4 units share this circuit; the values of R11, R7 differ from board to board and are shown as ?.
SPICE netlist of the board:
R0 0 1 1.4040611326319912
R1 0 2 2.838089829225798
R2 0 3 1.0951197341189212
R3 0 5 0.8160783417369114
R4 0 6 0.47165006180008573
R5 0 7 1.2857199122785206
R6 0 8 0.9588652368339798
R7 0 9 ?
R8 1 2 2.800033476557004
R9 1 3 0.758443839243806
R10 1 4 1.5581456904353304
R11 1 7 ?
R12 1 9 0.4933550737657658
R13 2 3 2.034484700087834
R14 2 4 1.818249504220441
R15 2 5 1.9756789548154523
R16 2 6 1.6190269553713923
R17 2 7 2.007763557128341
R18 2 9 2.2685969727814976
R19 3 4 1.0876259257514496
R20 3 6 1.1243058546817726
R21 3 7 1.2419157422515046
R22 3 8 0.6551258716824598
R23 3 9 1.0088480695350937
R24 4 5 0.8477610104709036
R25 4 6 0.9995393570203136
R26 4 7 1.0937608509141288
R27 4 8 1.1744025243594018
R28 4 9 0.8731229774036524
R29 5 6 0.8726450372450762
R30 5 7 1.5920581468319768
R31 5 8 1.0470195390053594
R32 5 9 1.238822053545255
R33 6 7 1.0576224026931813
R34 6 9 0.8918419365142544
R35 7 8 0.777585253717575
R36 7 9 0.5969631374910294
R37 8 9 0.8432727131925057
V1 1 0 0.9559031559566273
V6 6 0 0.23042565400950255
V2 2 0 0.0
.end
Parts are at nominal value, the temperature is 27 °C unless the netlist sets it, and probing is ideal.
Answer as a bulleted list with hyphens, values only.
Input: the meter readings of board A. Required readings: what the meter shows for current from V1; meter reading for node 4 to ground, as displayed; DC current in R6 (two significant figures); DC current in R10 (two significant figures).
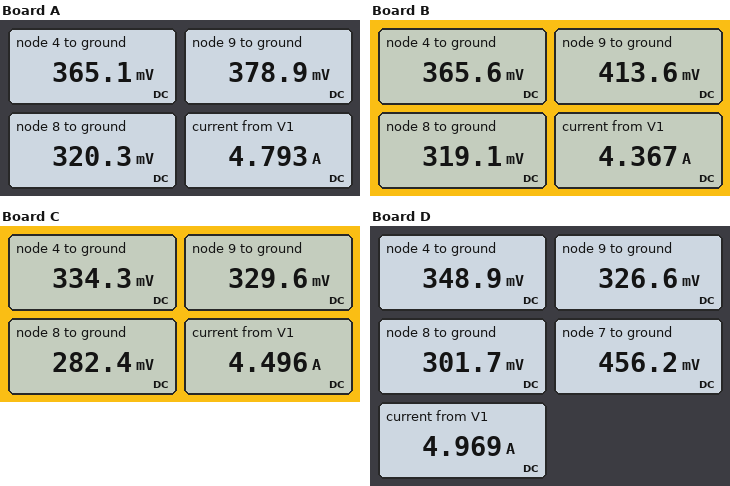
- 4.793 A
- 365.1 mV
- 330 mA
- 380 mA
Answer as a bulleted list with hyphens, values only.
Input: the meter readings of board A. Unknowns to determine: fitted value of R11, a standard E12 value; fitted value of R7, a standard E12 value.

- 0.33 Ω
- 0.47 Ω
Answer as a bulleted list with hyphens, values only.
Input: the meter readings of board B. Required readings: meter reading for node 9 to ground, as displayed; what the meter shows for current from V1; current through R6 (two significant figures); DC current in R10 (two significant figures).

- 413.6 mV
- 4.367 A
- 330 mA
- 380 mA
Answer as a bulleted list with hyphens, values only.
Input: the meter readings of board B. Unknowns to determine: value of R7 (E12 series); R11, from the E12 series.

- 1 Ω
- 0.47 Ω
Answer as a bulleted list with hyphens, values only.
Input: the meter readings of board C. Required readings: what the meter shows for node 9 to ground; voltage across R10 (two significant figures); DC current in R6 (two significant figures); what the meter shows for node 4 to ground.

- 329.6 mV
- 620 mV
- 290 mA
- 334.3 mV
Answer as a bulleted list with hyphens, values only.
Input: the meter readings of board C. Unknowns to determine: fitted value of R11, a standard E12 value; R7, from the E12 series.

- 0.56 Ω
- 0.33 Ω
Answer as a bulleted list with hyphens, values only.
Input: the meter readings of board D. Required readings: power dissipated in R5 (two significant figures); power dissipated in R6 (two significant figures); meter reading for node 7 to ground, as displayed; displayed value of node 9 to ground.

- 160 mW
- 95 mW
- 456.2 mV
- 326.6 mV
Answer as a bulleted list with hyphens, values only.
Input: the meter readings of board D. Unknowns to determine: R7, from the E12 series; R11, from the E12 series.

- 0.27 Ω
- 0.33 Ω
